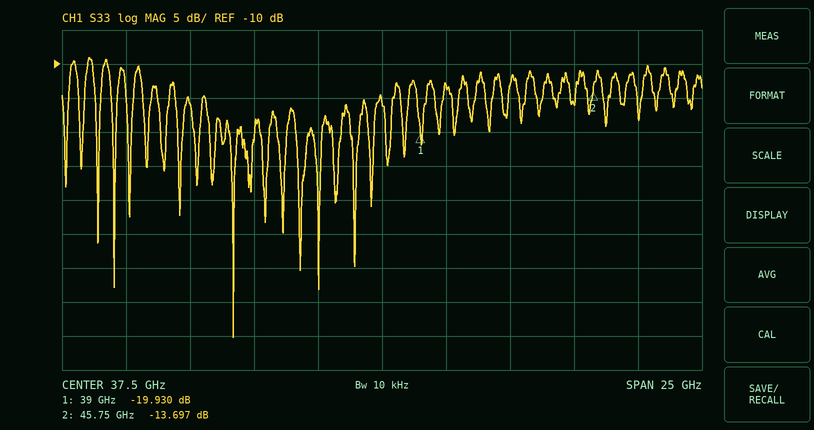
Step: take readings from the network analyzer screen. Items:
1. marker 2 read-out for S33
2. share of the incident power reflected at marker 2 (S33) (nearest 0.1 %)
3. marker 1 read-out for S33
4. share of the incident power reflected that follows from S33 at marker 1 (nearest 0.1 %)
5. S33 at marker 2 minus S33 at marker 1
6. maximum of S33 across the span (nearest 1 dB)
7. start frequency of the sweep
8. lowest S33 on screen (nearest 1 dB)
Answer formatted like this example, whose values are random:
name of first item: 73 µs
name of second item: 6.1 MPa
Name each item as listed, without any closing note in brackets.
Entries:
marker 2 read-out for S33: -13.697 dB
share of the incident power reflected at marker 2 (S33): 4.3 %
marker 1 read-out for S33: -19.930 dB
share of the incident power reflected that follows from S33 at marker 1: 1.0 %
S33 at marker 2 minus S33 at marker 1: 6.233 dB
maximum of S33 across the span: -9 dB
start frequency of the sweep: 25 GHz
lowest S33 on screen: -50 dB
